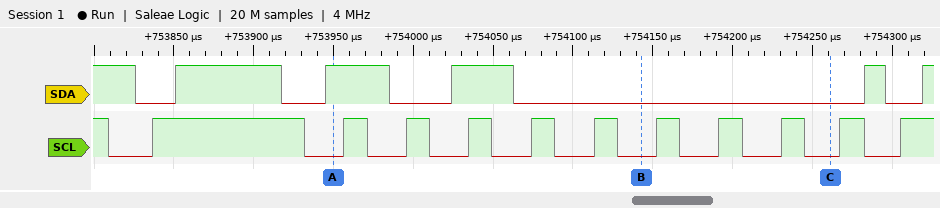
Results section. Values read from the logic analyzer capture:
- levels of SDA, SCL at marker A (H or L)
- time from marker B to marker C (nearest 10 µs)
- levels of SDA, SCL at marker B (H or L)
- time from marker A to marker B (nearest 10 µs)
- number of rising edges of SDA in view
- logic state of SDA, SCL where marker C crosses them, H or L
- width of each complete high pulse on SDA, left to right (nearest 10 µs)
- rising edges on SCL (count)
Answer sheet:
SDA=H, SCL=L
120 µs
SDA=L, SCL=L
190 µs
5
SDA=L, SCL=L
70 µs, 40 µs, 40 µs, 10 µs
11
